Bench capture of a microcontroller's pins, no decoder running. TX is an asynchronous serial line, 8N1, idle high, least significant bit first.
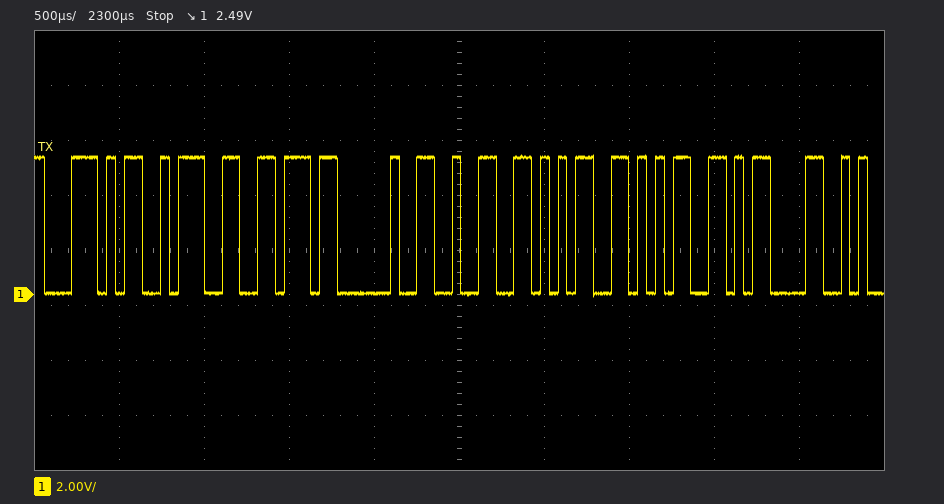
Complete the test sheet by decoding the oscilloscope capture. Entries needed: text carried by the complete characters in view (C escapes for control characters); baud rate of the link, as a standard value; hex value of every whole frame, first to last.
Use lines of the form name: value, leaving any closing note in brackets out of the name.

text carried by the complete characters in view: "\\:v 255\r"
baud rate of the link, as a standard value: 19200 baud
hex value of every whole frame, first to last: 0x5C 0x3A 0x76 0x20 0x32 0x35 0x35 0x0D
